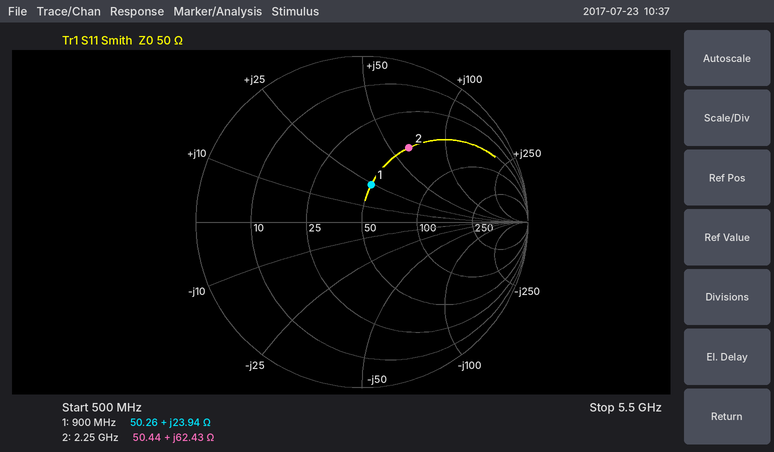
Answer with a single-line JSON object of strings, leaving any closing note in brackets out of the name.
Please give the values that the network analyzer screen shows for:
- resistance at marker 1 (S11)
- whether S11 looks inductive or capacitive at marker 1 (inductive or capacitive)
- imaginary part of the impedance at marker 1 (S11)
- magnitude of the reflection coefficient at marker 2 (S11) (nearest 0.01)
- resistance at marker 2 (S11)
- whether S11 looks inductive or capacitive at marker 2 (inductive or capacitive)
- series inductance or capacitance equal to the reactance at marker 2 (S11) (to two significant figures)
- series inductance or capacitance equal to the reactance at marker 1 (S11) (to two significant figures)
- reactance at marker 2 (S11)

{"resistance at marker 1": "50.26 Ω", "whether S11 looks inductive or capacitive at marker 1": "inductive", "imaginary part of the impedance at marker 1": "+23.94 Ω", "magnitude of the reflection coefficient at marker 2 (S11)": "0.53", "resistance at marker 2": "50.44 Ω", "whether S11 looks inductive or capacitive at marker 2": "inductive", "series inductance or capacitance equal to the reactance at marker 2 (S11)": "4.4 nH", "series inductance or capacitance equal to the reactance at marker 1 (S11)": "4.2 nH", "reactance at marker 2": "+62.43 Ω"}
